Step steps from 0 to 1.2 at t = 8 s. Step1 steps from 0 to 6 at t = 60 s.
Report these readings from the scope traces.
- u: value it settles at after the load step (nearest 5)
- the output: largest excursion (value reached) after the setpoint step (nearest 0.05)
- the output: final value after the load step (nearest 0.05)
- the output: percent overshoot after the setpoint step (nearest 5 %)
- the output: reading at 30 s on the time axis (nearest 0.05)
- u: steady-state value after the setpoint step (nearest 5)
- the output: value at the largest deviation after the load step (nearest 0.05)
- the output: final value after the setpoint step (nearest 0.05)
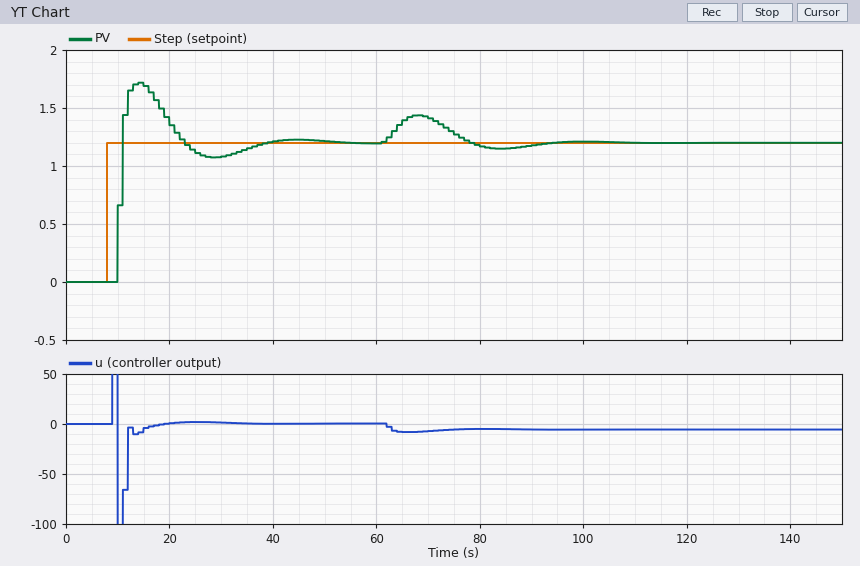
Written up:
-5
1.70
1.20
45 %
1.10
0
1.45
1.20
